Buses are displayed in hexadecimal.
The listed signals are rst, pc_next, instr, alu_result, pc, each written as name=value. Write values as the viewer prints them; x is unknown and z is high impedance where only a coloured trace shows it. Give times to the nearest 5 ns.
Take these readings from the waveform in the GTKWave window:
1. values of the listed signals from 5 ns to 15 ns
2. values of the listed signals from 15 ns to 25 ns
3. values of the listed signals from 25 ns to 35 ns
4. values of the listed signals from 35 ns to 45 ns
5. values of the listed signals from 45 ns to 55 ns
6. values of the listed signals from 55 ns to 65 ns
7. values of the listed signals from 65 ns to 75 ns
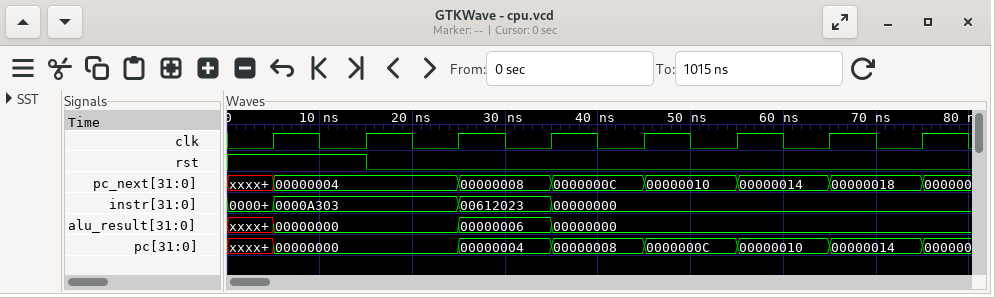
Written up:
rst=1, pc_next=00000004, instr=0000A303, alu_result=00000000, pc=00000000
rst=0, pc_next=00000004, instr=0000A303, alu_result=00000000, pc=00000000
rst=0, pc_next=00000008, instr=00612023, alu_result=00000006, pc=00000004
rst=0, pc_next=0000000C, instr=00000000, alu_result=00000000, pc=00000008
rst=0, pc_next=00000010, instr=00000000, alu_result=00000000, pc=0000000C
rst=0, pc_next=00000014, instr=00000000, alu_result=00000000, pc=00000010
rst=0, pc_next=00000018, instr=00000000, alu_result=00000000, pc=00000014
